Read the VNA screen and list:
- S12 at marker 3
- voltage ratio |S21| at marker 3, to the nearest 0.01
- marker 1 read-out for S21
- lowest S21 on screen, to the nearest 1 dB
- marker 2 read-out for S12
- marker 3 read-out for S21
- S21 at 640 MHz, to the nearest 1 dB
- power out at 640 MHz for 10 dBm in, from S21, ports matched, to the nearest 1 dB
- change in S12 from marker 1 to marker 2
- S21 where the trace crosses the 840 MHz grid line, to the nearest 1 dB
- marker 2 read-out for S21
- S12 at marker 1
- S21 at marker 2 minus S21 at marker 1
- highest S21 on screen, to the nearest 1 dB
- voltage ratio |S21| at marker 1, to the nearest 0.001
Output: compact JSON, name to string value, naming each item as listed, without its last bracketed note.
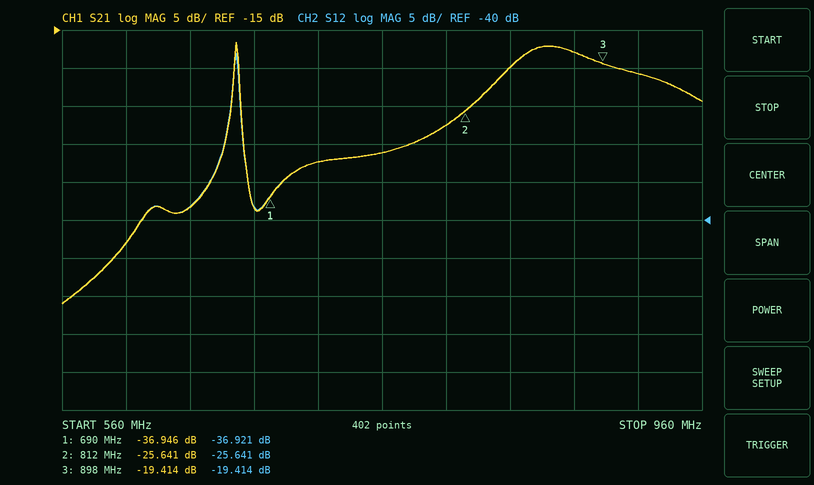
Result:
{"S12 at marker 3": "-19.414 dB", "voltage ratio |S21| at marker 3, to the nearest 0.01": "0.11", "marker 1 read-out for S21": "-36.946 dB", "lowest S21 on screen, to the nearest 1 dB": "-51 dB", "marker 2 read-out for S12": "-25.641 dB", "marker 3 read-out for S21": "-19.414 dB", "S21 at 640 MHz, to the nearest 1 dB": "-38 dB", "power out at 640 MHz for 10 dBm in, from S21, ports matched, to the nearest 1 dB": "-28 dBm", "change in S12 from marker 1 to marker 2": "11.280 dB", "S21 where the trace crosses the 840 MHz grid line, to the nearest 1 dB": "-20 dB", "marker 2 read-out for S21": "-25.641 dB", "S12 at marker 1": "-36.921 dB", "S21 at marker 2 minus S21 at marker 1": "11.305 dB", "highest S21 on screen, to the nearest 1 dB": "-17 dB", "voltage ratio |S21| at marker 1, to the nearest 0.001": "0.014"}
